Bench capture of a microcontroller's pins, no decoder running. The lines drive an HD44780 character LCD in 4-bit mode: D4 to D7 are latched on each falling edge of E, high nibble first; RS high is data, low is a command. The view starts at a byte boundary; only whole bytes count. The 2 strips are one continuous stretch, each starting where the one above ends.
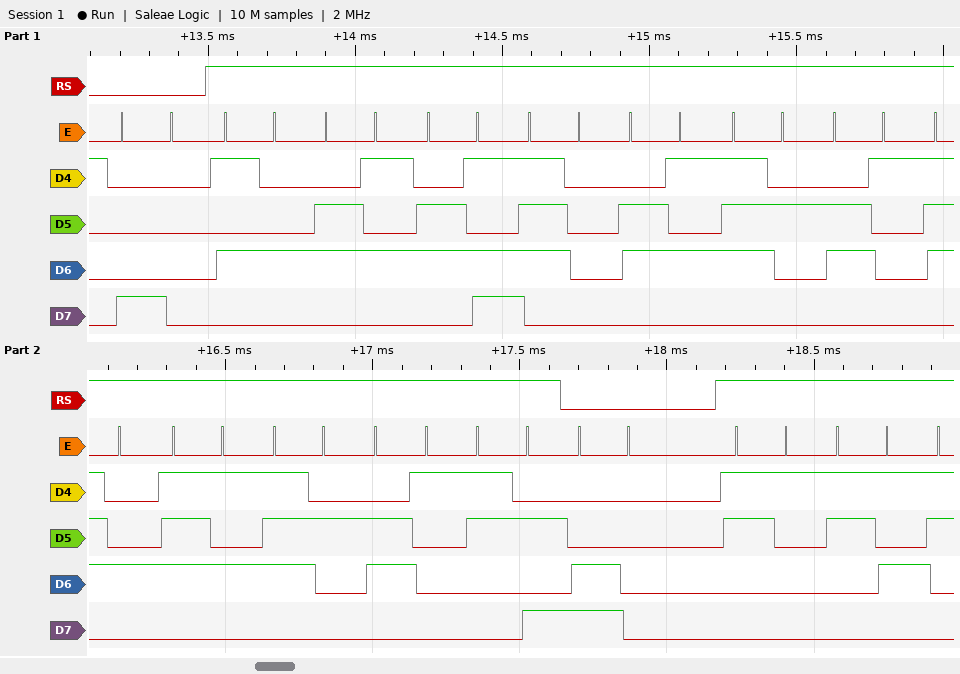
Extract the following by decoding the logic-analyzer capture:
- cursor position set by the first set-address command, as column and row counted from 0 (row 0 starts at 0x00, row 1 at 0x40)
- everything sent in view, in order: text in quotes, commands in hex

column 0, row 0
0x80 "Temperatura:" 0xC0 "15"
